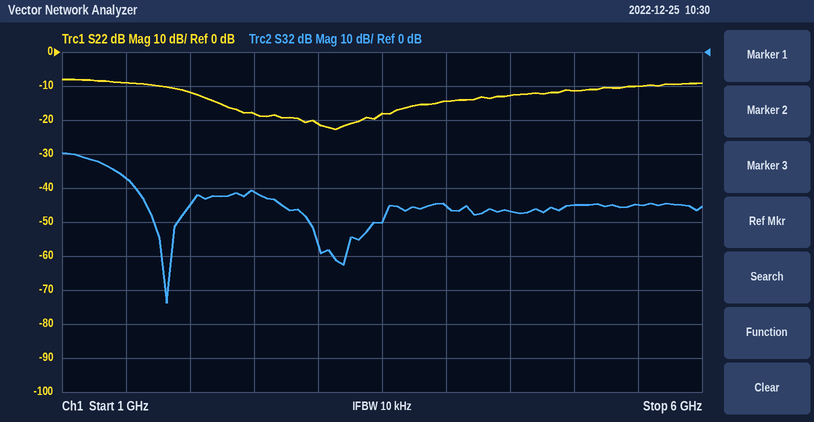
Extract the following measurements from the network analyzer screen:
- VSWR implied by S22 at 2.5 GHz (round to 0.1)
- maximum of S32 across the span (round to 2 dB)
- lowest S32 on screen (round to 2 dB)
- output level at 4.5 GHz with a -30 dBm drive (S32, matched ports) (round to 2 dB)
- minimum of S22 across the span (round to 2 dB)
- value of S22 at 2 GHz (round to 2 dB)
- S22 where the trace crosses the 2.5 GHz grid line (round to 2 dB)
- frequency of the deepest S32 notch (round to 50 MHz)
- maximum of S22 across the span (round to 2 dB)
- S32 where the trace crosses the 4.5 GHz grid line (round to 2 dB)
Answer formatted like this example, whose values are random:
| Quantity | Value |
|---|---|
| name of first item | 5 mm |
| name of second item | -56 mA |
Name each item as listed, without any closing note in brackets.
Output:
| Quantity | Value |
|---|---|
| VSWR implied by S22 at 2.5 GHz | 1.3 |
| maximum of S32 across the span | -30 dB |
| lowest S32 on screen | -74 dB |
| output level at 4.5 GHz with a -30 dBm drive (S32, matched ports) | -76 dBm |
| minimum of S22 across the span | -22 dB |
| value of S22 at 2 GHz | -12 dB |
| S22 where the trace crosses the 2.5 GHz grid line | -18 dB |
| frequency of the deepest S32 notch | 1.80 GHz |
| maximum of S22 across the span | -8 dB |
| S32 where the trace crosses the 4.5 GHz grid line | -46 dB |
